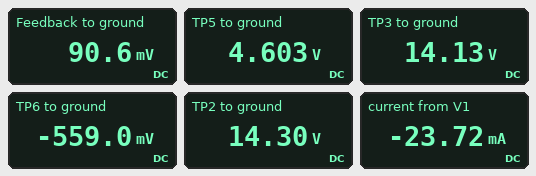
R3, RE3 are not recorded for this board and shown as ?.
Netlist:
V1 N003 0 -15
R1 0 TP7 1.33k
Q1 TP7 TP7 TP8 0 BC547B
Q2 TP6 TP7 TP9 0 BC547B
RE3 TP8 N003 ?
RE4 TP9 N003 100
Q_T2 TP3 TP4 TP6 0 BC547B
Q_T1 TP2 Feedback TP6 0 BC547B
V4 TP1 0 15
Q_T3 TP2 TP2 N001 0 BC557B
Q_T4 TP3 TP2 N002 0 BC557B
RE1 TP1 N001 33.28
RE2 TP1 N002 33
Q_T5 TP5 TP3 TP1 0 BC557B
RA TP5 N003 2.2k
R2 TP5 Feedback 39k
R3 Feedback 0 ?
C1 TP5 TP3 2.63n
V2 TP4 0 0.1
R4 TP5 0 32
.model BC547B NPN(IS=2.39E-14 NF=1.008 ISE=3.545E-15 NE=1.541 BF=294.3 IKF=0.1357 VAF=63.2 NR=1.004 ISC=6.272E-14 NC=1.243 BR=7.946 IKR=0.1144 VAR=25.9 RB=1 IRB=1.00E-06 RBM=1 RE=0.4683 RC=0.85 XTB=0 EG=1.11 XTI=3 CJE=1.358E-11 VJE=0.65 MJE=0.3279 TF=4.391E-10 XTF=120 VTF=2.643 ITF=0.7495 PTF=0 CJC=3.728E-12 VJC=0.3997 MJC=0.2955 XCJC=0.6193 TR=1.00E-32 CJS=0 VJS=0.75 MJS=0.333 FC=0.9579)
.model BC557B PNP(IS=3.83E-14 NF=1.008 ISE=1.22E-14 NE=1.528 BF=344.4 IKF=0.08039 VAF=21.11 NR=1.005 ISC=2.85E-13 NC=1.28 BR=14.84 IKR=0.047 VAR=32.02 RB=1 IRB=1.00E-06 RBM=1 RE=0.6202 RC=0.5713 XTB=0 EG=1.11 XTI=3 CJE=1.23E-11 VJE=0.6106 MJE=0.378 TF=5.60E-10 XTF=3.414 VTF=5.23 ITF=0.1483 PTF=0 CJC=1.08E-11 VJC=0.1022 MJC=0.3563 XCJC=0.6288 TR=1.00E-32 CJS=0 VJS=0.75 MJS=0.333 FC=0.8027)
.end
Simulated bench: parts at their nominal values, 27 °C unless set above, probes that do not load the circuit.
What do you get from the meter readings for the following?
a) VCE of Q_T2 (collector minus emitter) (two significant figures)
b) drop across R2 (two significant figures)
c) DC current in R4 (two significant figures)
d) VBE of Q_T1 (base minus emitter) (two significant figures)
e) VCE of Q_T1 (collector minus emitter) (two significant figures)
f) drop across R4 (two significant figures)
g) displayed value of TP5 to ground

15 V
4.5 V
140 mA
650 mV
15 V
4.6 V
4.603 V
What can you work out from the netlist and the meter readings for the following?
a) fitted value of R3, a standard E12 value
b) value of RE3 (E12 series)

820 Ω
39 Ω
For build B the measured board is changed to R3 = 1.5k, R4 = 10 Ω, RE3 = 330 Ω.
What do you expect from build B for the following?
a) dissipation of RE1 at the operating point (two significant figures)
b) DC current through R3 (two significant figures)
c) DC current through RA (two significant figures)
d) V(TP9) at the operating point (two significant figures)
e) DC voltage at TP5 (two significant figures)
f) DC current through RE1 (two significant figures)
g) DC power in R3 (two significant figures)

4.8 mW
61 µA
8.6 mA
-12 V
3.9 V
12 mA
5.5 µW
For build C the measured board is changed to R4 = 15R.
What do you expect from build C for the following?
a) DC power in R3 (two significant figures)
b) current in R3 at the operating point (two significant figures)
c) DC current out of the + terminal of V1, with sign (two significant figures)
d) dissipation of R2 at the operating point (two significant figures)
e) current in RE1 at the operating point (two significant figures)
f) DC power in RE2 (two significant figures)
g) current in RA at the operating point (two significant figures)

7.1 µW
93 µA
-23 mA
370 µW
1.3 mA
57 µW
8.6 mA
